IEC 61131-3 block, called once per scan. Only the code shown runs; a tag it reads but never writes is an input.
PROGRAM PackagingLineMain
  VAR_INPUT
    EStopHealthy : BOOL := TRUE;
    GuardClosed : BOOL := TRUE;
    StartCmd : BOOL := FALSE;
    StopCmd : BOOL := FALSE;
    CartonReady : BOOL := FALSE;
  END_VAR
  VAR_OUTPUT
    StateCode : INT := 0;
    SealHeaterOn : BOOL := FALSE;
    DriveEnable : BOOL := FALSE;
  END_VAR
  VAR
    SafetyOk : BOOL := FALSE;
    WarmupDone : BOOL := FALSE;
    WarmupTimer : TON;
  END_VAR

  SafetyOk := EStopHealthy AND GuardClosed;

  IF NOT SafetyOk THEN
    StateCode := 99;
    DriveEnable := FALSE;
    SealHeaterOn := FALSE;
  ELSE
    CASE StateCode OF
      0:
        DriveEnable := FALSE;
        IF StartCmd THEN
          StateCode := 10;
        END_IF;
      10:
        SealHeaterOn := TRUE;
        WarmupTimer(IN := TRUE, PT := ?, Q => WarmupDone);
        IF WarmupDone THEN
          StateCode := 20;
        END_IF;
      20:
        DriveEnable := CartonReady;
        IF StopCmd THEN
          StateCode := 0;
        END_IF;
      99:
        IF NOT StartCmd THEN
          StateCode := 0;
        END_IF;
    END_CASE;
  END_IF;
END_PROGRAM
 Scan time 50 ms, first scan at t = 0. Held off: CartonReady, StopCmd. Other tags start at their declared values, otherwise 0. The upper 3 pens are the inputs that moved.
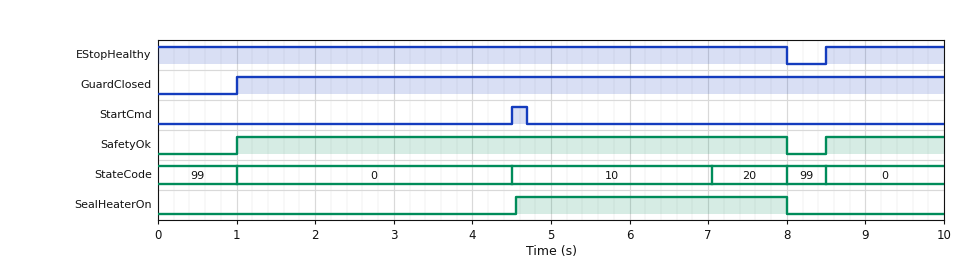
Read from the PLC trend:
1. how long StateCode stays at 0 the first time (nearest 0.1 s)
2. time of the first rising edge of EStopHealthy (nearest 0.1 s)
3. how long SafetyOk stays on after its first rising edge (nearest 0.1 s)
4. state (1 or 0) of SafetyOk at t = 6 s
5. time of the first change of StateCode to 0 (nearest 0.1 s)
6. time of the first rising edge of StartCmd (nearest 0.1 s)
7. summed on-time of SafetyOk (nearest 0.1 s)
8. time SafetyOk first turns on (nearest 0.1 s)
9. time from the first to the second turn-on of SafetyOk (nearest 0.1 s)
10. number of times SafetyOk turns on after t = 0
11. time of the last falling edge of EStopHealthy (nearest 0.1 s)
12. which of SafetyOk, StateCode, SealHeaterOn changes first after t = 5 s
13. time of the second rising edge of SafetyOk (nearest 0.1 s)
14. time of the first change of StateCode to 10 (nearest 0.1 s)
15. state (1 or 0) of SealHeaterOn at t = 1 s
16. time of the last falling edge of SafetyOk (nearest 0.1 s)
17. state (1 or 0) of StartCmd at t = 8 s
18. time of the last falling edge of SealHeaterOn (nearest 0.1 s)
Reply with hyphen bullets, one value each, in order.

- 3.5 s
- 8.5 s
- 7.0 s
- 1
- 1.0 s
- 4.5 s
- 8.5 s
- 1.0 s
- 7.5 s
- 2
- 8.0 s
- StateCode
- 8.5 s
- 4.5 s
- 0
- 8.0 s
- 0
- 8.0 s
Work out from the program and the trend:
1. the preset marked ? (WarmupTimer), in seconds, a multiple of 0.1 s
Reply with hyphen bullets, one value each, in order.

- 2.5 s
